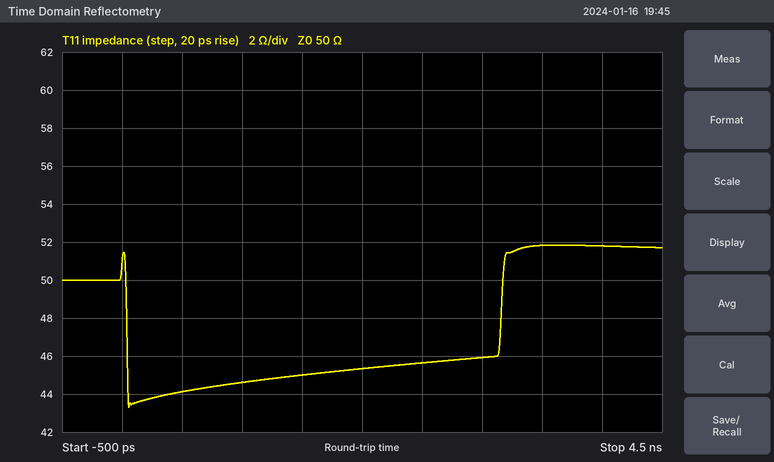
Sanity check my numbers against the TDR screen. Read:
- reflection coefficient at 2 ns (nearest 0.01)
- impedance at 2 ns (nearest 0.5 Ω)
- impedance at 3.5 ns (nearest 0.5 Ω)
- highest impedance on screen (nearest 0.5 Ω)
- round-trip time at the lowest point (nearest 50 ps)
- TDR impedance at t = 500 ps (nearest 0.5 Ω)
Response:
-0.05
45.5 Ω
52.0 Ω
52.0 Ω
50 ps
44.0 Ω
